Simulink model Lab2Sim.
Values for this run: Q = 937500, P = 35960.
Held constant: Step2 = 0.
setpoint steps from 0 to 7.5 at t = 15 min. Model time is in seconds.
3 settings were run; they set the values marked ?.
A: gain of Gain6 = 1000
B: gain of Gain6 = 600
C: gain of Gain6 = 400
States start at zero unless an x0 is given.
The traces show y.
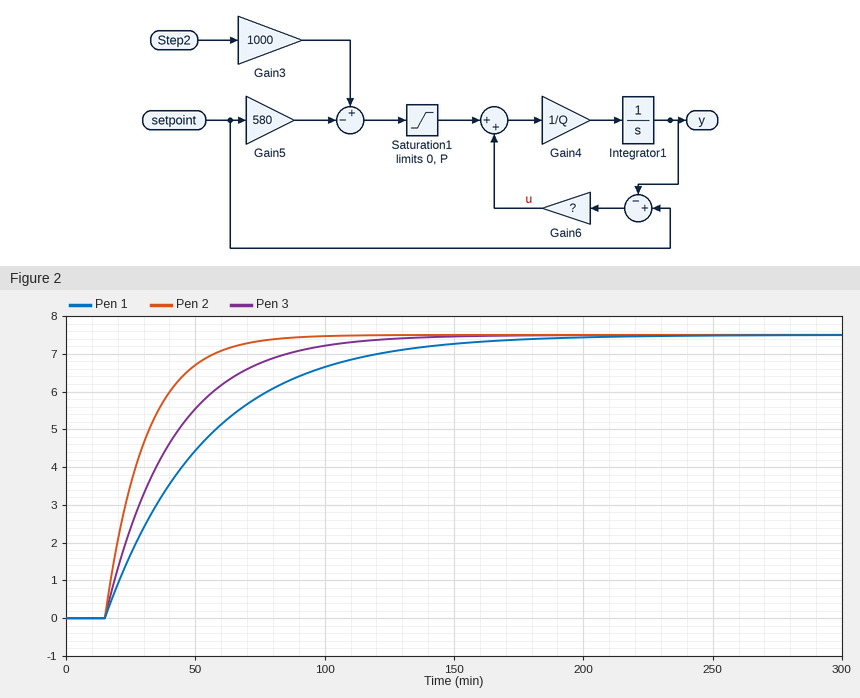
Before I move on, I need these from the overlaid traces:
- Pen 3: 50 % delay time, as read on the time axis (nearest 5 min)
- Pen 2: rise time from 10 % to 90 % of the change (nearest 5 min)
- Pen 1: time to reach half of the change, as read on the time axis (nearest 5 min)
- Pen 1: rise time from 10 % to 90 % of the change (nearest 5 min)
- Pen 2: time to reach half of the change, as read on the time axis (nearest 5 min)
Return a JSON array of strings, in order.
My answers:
["35 min", "35 min", "40 min", "85 min", "25 min"]
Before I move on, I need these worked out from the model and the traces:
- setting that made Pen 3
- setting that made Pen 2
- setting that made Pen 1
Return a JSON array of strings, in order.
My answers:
["B", "A", "C"]
